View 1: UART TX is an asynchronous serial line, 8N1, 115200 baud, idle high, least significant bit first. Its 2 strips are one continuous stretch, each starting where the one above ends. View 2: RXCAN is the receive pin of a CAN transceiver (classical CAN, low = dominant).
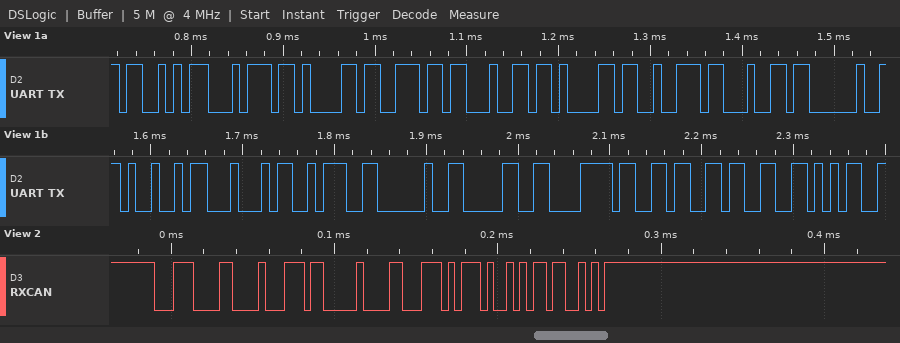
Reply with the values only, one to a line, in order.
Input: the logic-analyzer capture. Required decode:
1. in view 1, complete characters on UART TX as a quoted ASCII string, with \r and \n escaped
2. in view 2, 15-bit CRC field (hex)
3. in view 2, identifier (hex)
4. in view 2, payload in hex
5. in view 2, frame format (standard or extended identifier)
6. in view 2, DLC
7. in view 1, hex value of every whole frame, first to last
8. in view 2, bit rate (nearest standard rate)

"Standard ID: 0x635"
0x15B2
0x1C3
76 00 C7 5D
standard
4
53 74 61 6E 64 61 72 64 20 49 44 3A 20 30 78 36 33 35
250 kbit/s
